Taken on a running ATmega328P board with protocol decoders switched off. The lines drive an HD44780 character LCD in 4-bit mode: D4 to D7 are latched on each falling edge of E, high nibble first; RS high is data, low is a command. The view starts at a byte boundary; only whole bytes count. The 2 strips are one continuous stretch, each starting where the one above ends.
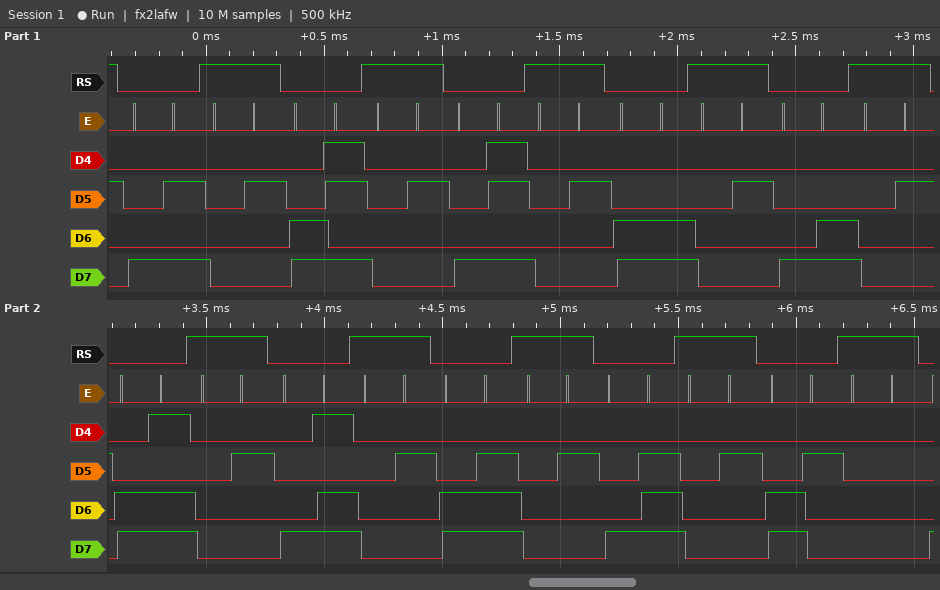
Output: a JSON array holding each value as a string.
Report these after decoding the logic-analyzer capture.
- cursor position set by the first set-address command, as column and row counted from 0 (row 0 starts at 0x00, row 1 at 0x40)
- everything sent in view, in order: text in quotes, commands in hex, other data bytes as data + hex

["column 10, row 0", "0x8A data 02 0xCB data 02 0x8B data 02 0xCC data 02 0x8C data 02 0xCD data 02 0x8D data 02 0xCE data 02 0x8E data 02 0xC2 data 00"]
